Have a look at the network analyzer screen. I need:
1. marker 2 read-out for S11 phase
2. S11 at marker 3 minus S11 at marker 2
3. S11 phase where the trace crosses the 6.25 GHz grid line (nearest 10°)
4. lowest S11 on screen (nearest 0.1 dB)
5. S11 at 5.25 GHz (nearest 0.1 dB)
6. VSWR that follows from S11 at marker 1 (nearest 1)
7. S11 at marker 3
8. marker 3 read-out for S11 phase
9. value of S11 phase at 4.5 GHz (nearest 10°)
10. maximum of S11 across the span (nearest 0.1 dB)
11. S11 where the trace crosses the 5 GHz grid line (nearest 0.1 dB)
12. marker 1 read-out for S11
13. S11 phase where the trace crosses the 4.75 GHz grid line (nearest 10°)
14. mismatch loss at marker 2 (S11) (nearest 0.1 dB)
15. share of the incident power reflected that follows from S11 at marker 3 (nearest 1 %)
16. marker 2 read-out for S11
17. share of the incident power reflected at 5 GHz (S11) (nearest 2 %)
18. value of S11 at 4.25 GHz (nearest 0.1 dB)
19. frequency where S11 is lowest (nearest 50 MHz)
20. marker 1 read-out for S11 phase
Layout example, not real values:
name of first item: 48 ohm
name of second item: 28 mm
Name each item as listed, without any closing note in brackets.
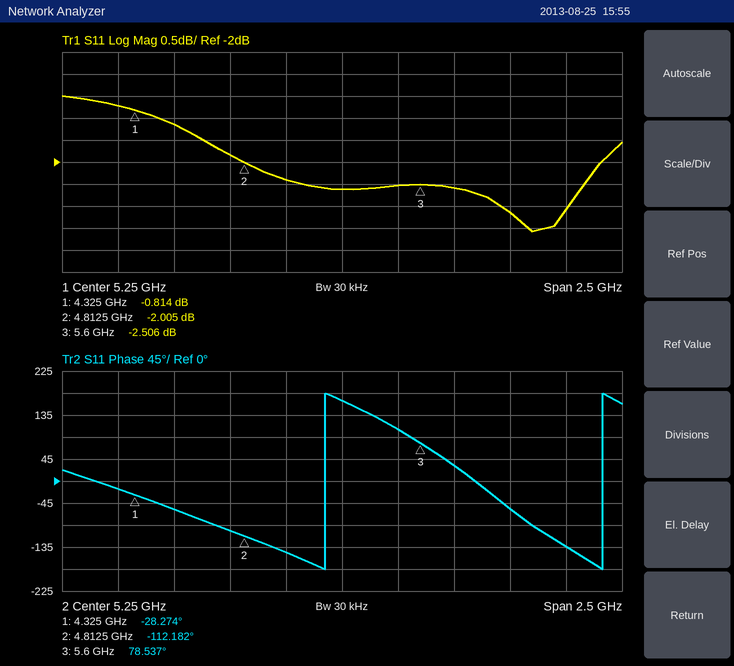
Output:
marker 2 read-out for S11 phase: -112.182°
S11 at marker 3 minus S11 at marker 2: -0.501 dB
S11 phase where the trace crosses the 6.25 GHz grid line: -130°
lowest S11 on screen: -3.6 dB
S11 at 5.25 GHz: -2.6 dB
VSWR that follows from S11 at marker 1: 21
S11 at marker 3: -2.506 dB
marker 3 read-out for S11 phase: 78.537°
value of S11 phase at 4.5 GHz: -60°
maximum of S11 across the span: -0.5 dB
S11 where the trace crosses the 5 GHz grid line: -2.4 dB
marker 1 read-out for S11: -0.814 dB
S11 phase where the trace crosses the 4.75 GHz grid line: -100°
mismatch loss at marker 2 (S11): 4.3 dB
share of the incident power reflected that follows from S11 at marker 3: 56 %
marker 2 read-out for S11: -2.005 dB
share of the incident power reflected at 5 GHz (S11): 58 %
value of S11 at 4.25 GHz: -0.7 dB
frequency where S11 is lowest: 6.10 GHz
marker 1 read-out for S11 phase: -28.274°
